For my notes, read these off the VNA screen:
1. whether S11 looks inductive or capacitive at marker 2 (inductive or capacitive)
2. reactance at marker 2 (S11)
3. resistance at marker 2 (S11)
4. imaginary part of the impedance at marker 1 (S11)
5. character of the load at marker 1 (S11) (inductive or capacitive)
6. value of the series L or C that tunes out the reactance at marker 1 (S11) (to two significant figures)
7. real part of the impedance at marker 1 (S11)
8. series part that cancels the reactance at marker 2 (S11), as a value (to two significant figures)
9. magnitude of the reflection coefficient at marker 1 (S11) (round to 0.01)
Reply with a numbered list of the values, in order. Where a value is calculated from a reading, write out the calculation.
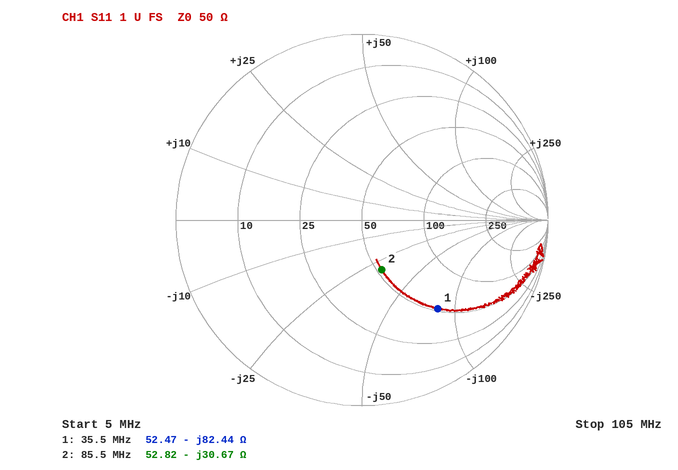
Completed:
1. capacitive
2. -30.67 Ω
3. 52.82 Ω
4. -82.44 Ω
5. capacitive
6. L = 82.44 Ω/(2π × 35.5 MHz) ≈ 370 nH
7. 52.47 Ω
8. L = 30.67 Ω/(2π × 85.5 MHz) ≈ 57 nH
9. 0.63
